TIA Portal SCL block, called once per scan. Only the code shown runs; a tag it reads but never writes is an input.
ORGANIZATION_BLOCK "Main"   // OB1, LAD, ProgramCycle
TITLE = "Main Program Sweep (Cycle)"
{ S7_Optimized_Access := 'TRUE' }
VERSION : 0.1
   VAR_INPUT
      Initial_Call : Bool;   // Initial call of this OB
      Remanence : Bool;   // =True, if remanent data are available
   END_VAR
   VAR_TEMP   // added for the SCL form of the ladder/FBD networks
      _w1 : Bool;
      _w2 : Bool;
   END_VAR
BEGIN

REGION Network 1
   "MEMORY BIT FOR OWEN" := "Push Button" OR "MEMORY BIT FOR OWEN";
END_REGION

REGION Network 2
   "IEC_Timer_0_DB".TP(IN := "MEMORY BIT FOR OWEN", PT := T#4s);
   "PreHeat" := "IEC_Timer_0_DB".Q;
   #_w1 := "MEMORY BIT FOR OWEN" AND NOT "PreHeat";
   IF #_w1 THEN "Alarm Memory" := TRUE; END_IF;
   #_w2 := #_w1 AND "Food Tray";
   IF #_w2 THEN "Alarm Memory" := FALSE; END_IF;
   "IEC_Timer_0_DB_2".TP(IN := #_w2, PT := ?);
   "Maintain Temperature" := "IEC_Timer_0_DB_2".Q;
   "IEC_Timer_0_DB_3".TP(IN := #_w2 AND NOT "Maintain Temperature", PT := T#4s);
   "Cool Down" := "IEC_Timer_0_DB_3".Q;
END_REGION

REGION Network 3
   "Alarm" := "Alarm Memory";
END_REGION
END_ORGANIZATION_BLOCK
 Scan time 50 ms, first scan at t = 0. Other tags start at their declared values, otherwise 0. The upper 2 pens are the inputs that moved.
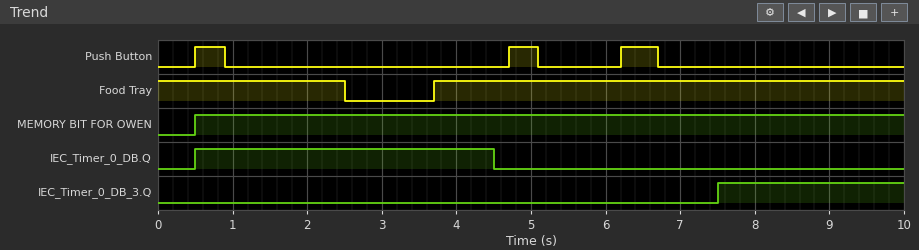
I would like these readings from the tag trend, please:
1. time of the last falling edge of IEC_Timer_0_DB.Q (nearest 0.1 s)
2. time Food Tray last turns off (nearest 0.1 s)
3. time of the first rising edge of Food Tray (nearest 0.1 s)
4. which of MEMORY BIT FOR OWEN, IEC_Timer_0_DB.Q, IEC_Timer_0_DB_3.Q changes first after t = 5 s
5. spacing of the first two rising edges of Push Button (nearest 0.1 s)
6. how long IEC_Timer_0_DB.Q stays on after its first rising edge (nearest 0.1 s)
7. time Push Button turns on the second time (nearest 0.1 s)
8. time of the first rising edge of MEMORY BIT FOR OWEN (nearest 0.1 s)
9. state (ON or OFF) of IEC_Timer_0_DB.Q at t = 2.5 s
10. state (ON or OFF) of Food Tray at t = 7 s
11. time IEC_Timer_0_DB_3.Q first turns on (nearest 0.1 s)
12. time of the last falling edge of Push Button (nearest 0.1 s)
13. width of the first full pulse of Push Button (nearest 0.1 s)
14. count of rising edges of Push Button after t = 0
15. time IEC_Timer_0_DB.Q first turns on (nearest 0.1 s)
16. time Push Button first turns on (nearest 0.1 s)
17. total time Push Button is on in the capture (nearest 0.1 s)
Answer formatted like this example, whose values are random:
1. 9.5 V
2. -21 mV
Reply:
1. 4.5 s
2. 2.5 s
3. 3.7 s
4. IEC_Timer_0_DB_3.Q
5. 4.2 s
6. 4.0 s
7. 4.7 s
8. 0.5 s
9. ON
10. ON
11. 7.5 s
12. 6.7 s
13. 0.4 s
14. 3
15. 0.5 s
16. 0.5 s
17. 1.3 s
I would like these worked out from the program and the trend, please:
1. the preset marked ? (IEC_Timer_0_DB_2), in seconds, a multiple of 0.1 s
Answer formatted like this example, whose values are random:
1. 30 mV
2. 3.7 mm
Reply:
1. 3.0 s
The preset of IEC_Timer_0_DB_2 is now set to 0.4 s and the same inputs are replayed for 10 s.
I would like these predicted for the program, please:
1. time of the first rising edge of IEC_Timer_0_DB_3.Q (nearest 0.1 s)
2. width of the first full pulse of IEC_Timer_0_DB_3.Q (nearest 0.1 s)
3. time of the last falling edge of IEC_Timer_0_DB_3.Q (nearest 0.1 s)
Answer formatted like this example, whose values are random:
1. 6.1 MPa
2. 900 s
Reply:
1. 4.9 s
2. 4.0 s
3. 8.9 s
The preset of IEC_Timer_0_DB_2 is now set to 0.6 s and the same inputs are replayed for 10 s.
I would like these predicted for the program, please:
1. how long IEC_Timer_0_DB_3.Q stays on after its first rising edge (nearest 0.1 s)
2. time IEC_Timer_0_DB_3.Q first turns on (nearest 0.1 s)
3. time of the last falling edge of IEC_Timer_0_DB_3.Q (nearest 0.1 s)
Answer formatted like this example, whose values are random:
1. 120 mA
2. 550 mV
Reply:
1. 4.0 s
2. 5.1 s
3. 9.1 s
